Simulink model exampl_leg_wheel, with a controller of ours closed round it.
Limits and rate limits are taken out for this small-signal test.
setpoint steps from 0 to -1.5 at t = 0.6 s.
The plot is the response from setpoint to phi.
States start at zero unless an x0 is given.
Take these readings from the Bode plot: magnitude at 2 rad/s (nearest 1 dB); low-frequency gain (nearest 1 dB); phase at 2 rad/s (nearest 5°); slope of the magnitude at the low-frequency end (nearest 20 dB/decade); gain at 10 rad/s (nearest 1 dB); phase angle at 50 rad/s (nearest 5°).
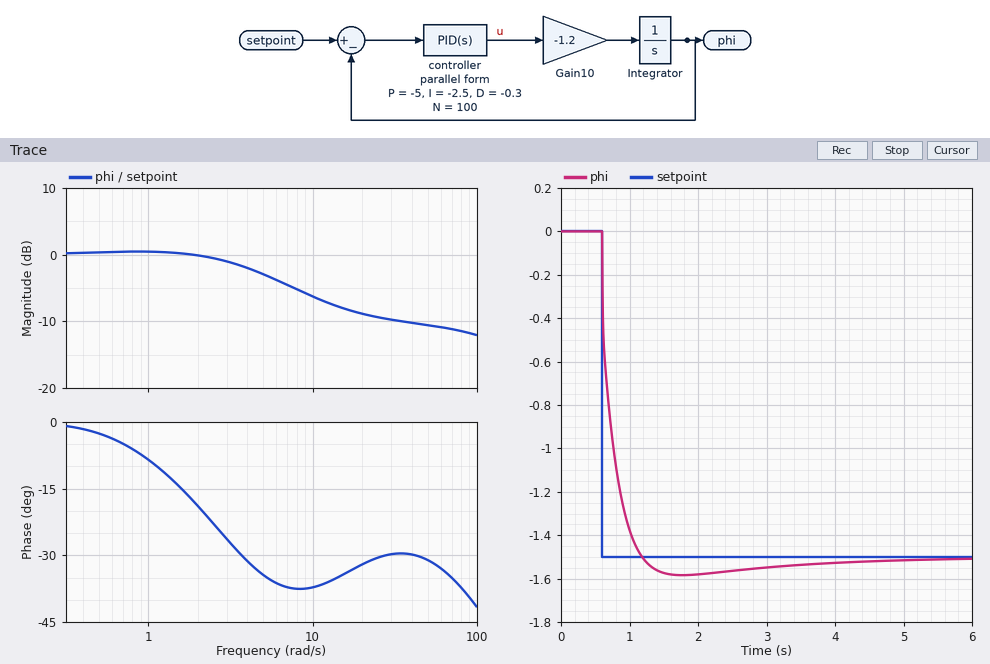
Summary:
0 dB
0 dB
-20°
0 dB/decade
-6 dB
-30°
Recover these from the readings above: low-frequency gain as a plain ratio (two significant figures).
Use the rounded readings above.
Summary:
1.0
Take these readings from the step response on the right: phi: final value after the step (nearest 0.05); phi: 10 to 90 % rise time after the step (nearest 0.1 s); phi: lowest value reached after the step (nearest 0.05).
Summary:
-1.50
0.4 s
-1.60
